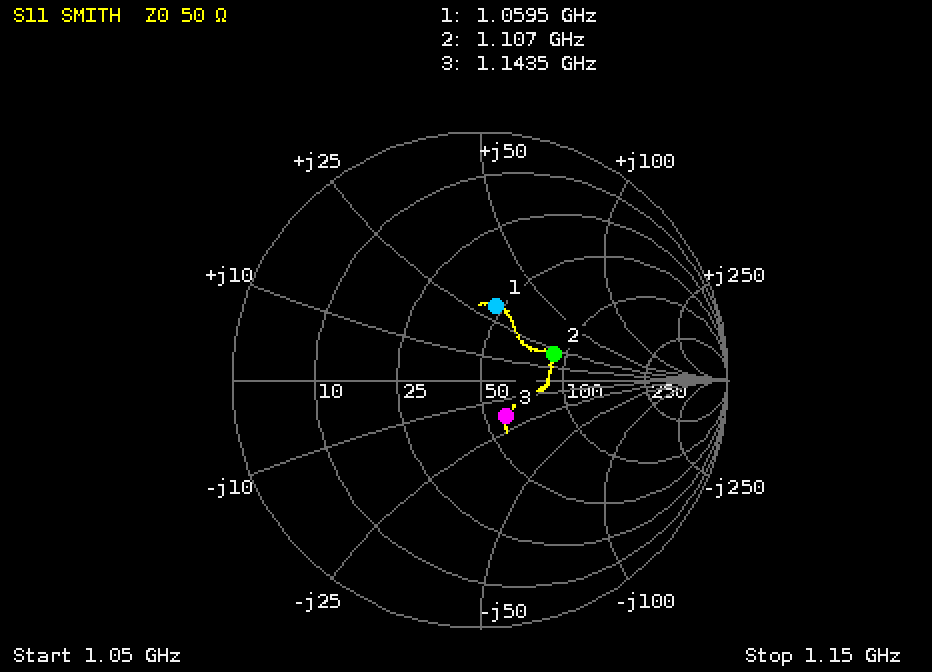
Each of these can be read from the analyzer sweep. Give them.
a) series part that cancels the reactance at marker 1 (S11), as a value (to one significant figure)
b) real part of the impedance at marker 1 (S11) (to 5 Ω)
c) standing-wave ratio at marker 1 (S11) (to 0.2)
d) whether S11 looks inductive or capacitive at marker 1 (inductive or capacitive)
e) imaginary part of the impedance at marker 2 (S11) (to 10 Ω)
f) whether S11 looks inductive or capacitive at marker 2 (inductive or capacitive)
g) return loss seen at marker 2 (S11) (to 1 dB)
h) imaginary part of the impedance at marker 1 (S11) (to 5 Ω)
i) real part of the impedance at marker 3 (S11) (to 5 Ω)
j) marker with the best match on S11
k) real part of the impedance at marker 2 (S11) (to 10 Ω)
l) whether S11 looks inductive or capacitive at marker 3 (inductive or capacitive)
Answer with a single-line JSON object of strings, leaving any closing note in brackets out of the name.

{"series part that cancels the reactance at marker 1 (S11), as a value": "5 pF", "real part of the impedance at marker 1 (S11)": "45 Ω", "standing-wave ratio at marker 1 (S11)": "1.8", "whether S11 looks inductive or capacitive at marker 1": "inductive", "imaginary part of the impedance at marker 2 (S11)": "+20 Ω", "whether S11 looks inductive or capacitive at marker 2": "inductive", "return loss seen at marker 2 (S11)": "10 dB", "imaginary part of the impedance at marker 1 (S11)": "+30 Ω", "real part of the impedance at marker 3 (S11)": "60 Ω", "marker with the best match on S11": "marker 3", "real part of the impedance at marker 2 (S11)": "90 Ω", "whether S11 looks inductive or capacitive at marker 3": "capacitive"}
